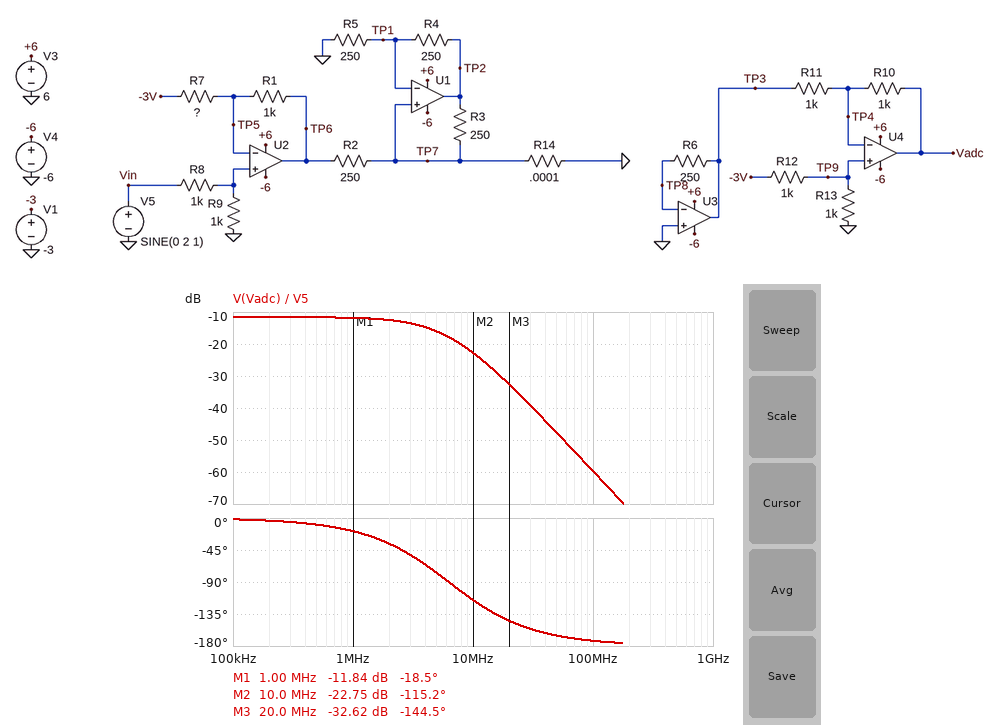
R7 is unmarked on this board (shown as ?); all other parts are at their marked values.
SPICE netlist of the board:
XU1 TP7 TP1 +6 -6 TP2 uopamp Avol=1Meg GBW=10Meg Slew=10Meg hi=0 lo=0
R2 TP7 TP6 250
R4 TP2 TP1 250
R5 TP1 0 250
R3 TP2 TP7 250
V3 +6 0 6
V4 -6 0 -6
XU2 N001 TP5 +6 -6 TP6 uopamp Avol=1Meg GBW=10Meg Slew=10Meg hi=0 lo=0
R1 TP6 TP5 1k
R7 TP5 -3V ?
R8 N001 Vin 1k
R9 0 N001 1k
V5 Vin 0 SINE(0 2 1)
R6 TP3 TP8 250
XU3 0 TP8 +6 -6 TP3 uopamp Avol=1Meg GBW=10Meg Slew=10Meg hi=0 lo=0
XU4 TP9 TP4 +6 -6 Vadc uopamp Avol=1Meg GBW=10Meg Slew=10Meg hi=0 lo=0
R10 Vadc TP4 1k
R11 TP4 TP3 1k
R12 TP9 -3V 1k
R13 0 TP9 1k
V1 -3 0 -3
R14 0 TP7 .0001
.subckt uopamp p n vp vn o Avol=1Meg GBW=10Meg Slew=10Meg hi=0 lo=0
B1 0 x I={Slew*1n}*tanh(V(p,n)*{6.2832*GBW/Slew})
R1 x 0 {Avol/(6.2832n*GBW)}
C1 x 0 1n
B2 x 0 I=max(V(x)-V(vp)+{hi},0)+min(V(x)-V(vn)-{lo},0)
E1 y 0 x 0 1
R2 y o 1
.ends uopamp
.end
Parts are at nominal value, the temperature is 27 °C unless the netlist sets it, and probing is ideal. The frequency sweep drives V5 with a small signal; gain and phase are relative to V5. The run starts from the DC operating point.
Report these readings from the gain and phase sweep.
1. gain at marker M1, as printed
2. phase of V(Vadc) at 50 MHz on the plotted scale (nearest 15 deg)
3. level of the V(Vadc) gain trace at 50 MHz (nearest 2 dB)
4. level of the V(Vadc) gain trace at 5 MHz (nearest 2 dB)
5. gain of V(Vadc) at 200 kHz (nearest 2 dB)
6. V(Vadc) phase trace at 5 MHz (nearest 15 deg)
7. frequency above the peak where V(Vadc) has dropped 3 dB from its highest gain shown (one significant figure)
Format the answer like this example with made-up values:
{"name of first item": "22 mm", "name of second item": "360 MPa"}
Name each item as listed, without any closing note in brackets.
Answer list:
{"gain at marker M1, as printed": "-11.84 dB", "phase of V(Vadc) at 50 MHz on the plotted scale": "-165 deg", "level of the V(Vadc) gain trace at 50 MHz": "-48 dB", "level of the V(Vadc) gain trace at 5 MHz": "-16 dB", "gain of V(Vadc) at 200 kHz": "-12 dB", "V(Vadc) phase trace at 5 MHz": "-75 deg", "frequency above the peak where V(Vadc) has dropped 3 dB from its highest gain shown": "4 MHz"}
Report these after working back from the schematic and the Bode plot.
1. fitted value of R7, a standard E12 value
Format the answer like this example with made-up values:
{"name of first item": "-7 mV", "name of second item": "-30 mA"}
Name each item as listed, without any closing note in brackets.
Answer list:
{"fitted value of R7, a standard E12 value": "1.8 kΩ"}
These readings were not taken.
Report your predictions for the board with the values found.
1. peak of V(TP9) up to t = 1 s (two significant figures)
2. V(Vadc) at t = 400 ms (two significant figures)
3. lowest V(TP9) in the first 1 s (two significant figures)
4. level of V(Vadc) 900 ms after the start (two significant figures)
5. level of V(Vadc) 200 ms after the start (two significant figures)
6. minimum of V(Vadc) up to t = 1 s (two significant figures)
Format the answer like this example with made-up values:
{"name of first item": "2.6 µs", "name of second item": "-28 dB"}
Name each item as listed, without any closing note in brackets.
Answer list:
{"peak of V(TP9) up to t = 1 s": "260 mV", "V(Vadc) at t = 400 ms": "310 mV", "lowest V(TP9) in the first 1 s": "-260 mV", "level of V(Vadc) 900 ms after the start": "-310 mV", "level of V(Vadc) 200 ms after the start": "500 mV", "minimum of V(Vadc) up to t = 1 s": "-530 mV"}
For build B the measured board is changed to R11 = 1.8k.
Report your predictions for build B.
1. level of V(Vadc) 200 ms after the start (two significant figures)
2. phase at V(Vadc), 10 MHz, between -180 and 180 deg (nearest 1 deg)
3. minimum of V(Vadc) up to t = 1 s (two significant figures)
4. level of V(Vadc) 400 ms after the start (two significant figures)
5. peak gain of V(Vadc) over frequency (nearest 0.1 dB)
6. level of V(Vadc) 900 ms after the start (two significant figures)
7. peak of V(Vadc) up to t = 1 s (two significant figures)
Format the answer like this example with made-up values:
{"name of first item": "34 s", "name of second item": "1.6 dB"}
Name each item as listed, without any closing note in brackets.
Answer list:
{"level of V(Vadc) 200 ms after the start": "390 mV", "phase at V(Vadc), 10 MHz, between -180 and 180 deg": "-109 deg", "minimum of V(Vadc) up to t = 1 s": "-410 mV", "level of V(Vadc) 400 ms after the start": "240 mV", "peak gain of V(Vadc) over frequency": "-13.8 dB", "level of V(Vadc) 900 ms after the start": "-240 mV", "peak of V(Vadc) up to t = 1 s": "410 mV"}
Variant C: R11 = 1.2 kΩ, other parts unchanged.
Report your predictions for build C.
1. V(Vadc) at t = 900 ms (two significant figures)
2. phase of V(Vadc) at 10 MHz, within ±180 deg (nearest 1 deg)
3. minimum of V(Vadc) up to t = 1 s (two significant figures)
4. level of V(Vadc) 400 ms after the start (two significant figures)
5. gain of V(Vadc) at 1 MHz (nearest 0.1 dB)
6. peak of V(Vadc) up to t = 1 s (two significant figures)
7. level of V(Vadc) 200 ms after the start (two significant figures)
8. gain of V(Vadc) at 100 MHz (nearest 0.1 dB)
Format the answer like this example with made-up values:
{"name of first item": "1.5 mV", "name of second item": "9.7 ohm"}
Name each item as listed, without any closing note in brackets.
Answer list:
{"V(Vadc) at t = 900 ms": "-280 mV", "phase of V(Vadc) at 10 MHz, within ±180 deg": "-113 deg", "minimum of V(Vadc) up to t = 1 s": "-480 mV", "level of V(Vadc) 400 ms after the start": "280 mV", "gain of V(Vadc) at 1 MHz": "-12.6 dB", "peak of V(Vadc) up to t = 1 s": "480 mV", "level of V(Vadc) 200 ms after the start": "460 mV", "gain of V(Vadc) at 100 MHz": "-59.7 dB"}
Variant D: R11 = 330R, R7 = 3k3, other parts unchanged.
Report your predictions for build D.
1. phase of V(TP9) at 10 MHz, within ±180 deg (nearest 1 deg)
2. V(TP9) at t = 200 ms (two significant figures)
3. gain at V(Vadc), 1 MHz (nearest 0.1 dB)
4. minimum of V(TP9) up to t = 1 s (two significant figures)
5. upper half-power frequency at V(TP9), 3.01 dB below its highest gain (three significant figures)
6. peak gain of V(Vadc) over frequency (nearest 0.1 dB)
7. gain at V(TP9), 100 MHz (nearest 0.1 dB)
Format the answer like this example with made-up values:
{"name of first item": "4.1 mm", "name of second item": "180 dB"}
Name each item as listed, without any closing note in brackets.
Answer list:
{"phase of V(TP9) at 10 MHz, within ±180 deg": "-50 deg", "V(TP9) at t = 200 ms": "180 mV", "gain at V(Vadc), 1 MHz": "-9.1 dB", "minimum of V(TP9) up to t = 1 s": "-190 mV", "upper half-power frequency at V(TP9), 3.01 dB below its highest gain": "8.38 MHz", "peak gain of V(Vadc) over frequency": "-8.4 dB", "gain at V(TP9), 100 MHz": "-42.1 dB"}
